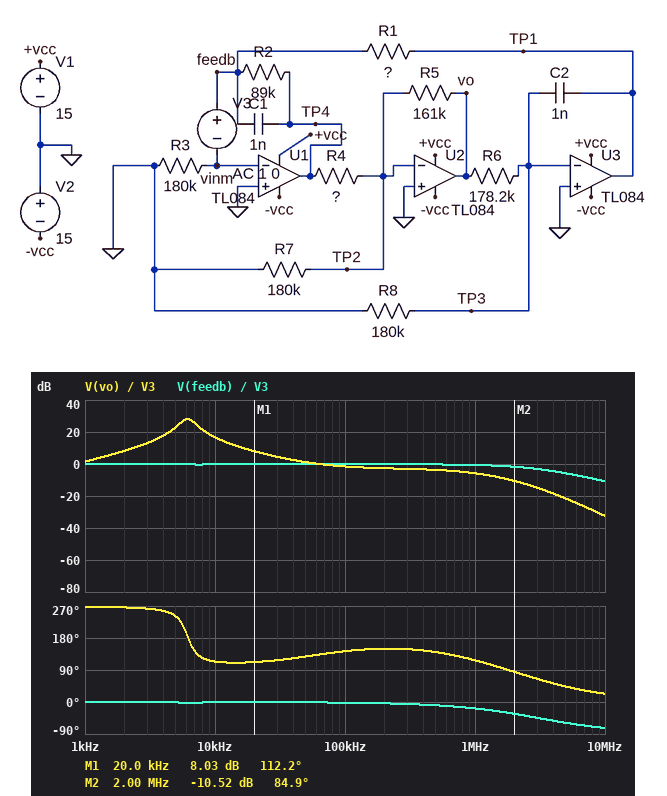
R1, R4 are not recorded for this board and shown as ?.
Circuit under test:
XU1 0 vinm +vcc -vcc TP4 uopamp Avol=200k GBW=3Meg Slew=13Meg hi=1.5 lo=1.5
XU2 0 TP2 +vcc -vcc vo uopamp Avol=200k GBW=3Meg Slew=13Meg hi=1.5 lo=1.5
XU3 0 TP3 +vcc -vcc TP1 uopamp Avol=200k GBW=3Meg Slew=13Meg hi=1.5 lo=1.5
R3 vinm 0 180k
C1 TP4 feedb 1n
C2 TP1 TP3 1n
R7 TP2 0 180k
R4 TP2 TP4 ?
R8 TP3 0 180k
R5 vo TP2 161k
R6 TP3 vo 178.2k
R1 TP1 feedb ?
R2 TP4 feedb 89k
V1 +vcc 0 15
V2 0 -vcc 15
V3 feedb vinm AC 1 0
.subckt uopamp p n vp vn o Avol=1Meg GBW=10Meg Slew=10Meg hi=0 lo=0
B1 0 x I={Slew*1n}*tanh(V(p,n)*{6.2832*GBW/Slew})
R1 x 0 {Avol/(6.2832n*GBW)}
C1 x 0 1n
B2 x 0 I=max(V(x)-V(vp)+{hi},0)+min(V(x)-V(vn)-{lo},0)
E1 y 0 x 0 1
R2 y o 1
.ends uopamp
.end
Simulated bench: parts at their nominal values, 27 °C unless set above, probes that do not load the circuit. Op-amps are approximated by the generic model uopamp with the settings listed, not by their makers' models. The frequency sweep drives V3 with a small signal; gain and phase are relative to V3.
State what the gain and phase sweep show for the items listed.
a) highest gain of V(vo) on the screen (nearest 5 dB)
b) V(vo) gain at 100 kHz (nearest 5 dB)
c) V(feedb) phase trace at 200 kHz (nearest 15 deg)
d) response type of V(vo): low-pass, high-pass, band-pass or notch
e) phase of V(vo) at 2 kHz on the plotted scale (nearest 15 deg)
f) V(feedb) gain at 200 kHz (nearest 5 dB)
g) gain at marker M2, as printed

30 dB
0 dB
0 deg
band-pass
270 deg
0 dB
-10.52 dB
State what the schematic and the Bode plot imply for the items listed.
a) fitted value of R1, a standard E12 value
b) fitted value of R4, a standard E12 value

2.7 kΩ
220 kΩ
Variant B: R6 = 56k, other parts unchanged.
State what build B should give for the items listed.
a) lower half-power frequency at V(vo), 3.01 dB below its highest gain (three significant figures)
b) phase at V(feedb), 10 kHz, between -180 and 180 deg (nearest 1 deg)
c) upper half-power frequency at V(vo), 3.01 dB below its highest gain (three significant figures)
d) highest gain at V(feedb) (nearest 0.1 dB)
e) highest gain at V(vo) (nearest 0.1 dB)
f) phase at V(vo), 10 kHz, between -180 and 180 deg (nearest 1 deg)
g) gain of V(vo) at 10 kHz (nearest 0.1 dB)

10.2 kHz
-2 deg
11.8 kHz
0.7 dB
29.0 dB
-119 deg
24.8 dB
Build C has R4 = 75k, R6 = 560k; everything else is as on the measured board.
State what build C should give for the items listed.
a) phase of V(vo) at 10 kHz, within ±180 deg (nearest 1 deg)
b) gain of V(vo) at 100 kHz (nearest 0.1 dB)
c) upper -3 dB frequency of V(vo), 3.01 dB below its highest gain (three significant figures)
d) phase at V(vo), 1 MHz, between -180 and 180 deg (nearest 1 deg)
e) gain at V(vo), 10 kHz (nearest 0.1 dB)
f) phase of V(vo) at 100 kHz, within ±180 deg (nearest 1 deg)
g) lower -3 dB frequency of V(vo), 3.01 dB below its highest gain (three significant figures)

113 deg
7.8 dB
6.84 kHz
105 deg
25.7 dB
140 deg
5.16 kHz
